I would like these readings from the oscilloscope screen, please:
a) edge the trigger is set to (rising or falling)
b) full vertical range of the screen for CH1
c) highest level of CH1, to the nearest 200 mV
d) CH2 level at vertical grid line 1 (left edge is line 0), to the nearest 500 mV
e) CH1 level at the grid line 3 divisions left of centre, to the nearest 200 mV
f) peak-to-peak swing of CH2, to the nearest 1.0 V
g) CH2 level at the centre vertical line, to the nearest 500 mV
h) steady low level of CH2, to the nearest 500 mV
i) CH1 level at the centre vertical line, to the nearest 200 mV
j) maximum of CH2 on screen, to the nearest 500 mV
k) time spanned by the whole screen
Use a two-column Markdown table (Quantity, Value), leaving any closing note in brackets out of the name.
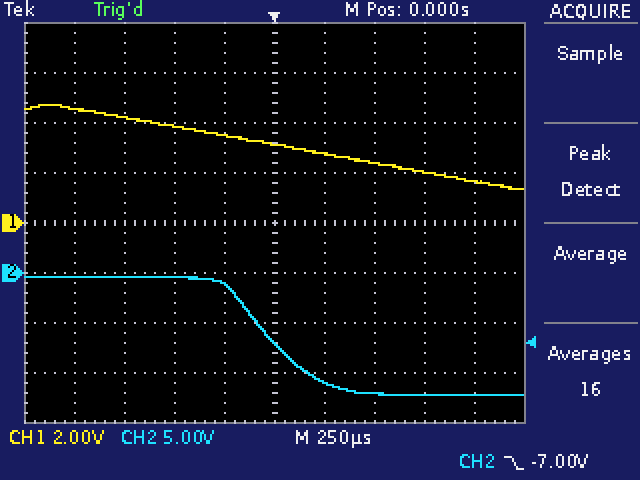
| Quantity | Value |
|---|---|
| edge the trigger is set to | falling |
| full vertical range of the screen for CH1 | 16 V |
| highest level of CH1, to the nearest 200 mV | 4.8 V |
| CH2 level at vertical grid line 1 (left edge is line 0), to the nearest 500 mV | -500 mV |
| CH1 level at the grid line 3 divisions left of centre, to the nearest 200 mV | 4.2 V |
| peak-to-peak swing of CH2, to the nearest 1.0 V | 12.0 V |
| CH2 level at the centre vertical line, to the nearest 500 mV | -7.0 V |
| steady low level of CH2, to the nearest 500 mV | -12.0 V |
| CH1 level at the centre vertical line, to the nearest 200 mV | 3.2 V |
| maximum of CH2 on screen, to the nearest 500 mV | -500 mV |
| time spanned by the whole screen | 2.5 ms |
